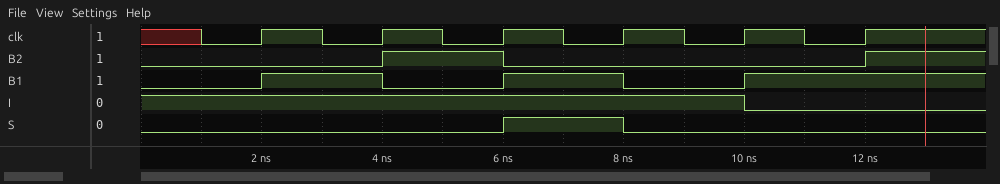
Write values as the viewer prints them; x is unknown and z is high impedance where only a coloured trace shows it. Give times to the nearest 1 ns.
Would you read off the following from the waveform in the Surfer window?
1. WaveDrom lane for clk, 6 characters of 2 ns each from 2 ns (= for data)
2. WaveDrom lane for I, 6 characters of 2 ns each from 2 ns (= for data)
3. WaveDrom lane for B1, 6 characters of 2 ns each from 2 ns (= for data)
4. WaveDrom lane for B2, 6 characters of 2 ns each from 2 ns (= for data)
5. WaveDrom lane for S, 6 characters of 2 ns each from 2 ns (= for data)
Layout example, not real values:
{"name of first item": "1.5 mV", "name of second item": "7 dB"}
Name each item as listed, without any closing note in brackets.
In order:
{"WaveDrom lane for clk, 6 characters of 2 ns each from 2 ns": "{name: 'clk', wave: 'p.....'}", "WaveDrom lane for I, 6 characters of 2 ns each from 2 ns": "{name: 'I', wave: '1...0.'}", "WaveDrom lane for B1, 6 characters of 2 ns each from 2 ns": "{name: 'B1', wave: '10101.'}", "WaveDrom lane for B2, 6 characters of 2 ns each from 2 ns": "{name: 'B2', wave: '010..1'}", "WaveDrom lane for S, 6 characters of 2 ns each from 2 ns": "{name: 'S', wave: '0.10..'}"}
